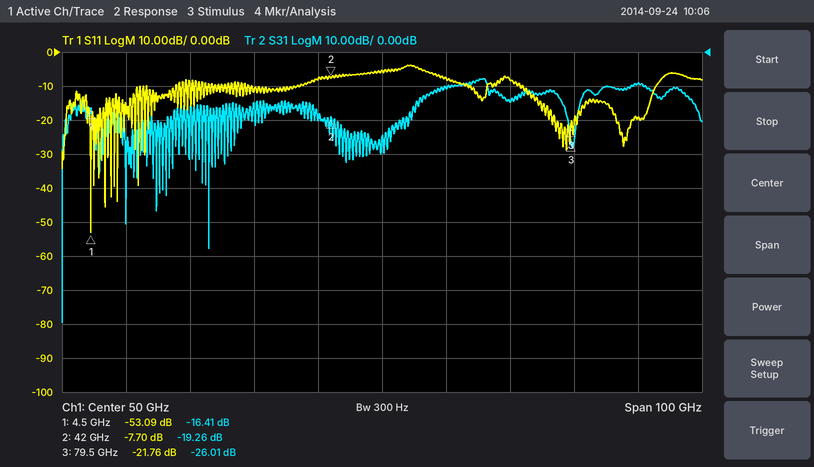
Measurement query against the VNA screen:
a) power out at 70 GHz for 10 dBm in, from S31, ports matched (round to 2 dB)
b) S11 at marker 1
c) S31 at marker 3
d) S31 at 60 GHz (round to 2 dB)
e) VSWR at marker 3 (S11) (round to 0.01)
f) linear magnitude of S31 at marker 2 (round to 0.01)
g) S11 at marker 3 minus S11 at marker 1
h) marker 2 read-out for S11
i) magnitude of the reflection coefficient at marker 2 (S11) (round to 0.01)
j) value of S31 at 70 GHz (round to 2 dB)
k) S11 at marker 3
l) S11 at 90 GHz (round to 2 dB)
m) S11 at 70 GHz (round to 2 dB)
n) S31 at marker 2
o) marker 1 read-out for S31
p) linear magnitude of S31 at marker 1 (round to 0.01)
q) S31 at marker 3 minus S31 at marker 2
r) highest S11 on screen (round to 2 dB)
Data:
-4 dBm
-53.09 dB
-26.01 dB
-10 dB
1.18
0.11
31.33 dB
-7.70 dB
0.41
-14 dB
-21.76 dB
-20 dB
-8 dB
-19.26 dB
-16.41 dB
0.15
-6.75 dB
-4 dB
